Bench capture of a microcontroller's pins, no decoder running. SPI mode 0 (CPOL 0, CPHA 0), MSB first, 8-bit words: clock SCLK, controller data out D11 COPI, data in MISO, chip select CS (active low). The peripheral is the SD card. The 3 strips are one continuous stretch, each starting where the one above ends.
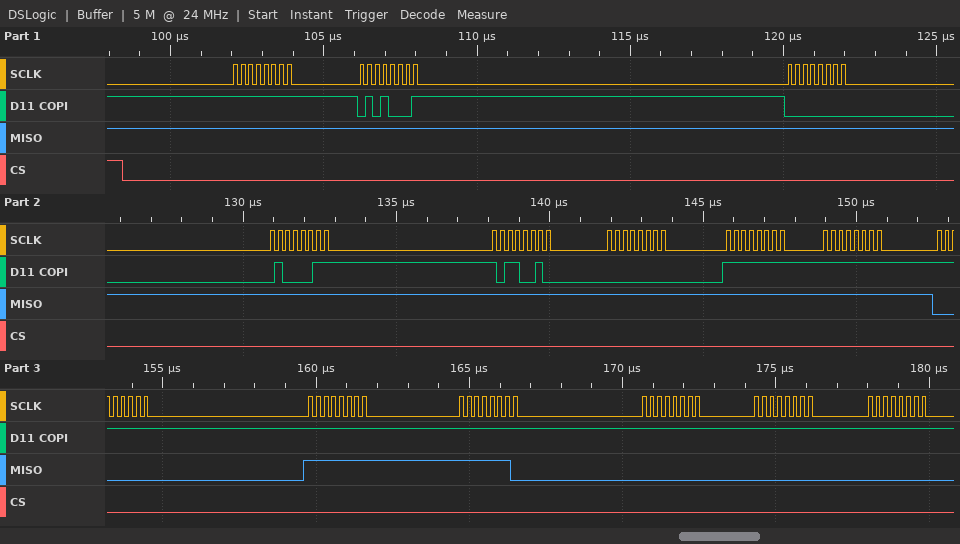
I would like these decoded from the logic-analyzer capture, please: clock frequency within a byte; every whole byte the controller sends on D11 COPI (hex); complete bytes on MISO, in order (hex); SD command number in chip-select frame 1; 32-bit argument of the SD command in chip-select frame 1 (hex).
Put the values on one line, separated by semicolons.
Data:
4 MHz; 0xFF 0x51 0x00 0x43 0xB2 0x00 0xFF 0xFF 0xFF 0xFF 0xFF 0xFF 0xFF 0xFF; 0xFF 0xFF 0xFF 0xFF 0xFF 0xFF 0xFF 0xFF 0x00 0xFF 0xFE 0x00 0x00 0x00; CMD17; 0x0043B200
